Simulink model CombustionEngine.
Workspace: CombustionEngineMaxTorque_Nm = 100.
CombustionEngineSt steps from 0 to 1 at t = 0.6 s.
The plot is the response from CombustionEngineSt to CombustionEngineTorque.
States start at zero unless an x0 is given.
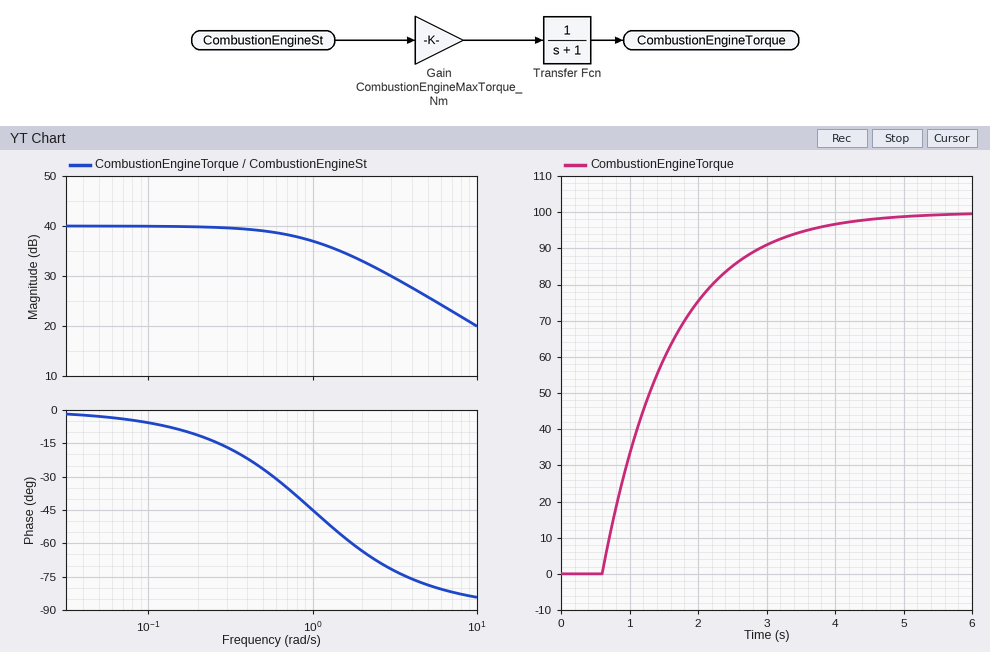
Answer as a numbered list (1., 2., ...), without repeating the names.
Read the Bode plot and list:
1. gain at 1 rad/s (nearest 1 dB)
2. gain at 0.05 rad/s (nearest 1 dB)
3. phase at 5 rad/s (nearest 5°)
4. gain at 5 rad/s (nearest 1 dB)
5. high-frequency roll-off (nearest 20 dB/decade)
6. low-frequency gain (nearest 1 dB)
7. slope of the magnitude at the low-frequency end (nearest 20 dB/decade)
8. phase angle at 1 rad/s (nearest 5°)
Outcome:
1. 37 dB
2. 40 dB
3. -80°
4. 26 dB
5. -20 dB/decade
6. 40 dB
7. 0 dB/decade
8. -45°
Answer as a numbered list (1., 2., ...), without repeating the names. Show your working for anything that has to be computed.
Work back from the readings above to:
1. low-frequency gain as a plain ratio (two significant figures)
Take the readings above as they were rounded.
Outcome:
1. 10^(40 / 20) = 100
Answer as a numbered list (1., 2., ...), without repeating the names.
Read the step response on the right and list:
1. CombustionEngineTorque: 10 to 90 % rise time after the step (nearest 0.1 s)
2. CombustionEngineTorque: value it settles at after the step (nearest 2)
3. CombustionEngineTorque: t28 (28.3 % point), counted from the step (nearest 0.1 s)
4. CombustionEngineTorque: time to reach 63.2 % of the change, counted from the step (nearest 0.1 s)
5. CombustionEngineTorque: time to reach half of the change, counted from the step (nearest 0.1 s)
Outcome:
1. 2.2 s
2. 100
3. 0.3 s
4. 1.0 s
5. 0.7 s
